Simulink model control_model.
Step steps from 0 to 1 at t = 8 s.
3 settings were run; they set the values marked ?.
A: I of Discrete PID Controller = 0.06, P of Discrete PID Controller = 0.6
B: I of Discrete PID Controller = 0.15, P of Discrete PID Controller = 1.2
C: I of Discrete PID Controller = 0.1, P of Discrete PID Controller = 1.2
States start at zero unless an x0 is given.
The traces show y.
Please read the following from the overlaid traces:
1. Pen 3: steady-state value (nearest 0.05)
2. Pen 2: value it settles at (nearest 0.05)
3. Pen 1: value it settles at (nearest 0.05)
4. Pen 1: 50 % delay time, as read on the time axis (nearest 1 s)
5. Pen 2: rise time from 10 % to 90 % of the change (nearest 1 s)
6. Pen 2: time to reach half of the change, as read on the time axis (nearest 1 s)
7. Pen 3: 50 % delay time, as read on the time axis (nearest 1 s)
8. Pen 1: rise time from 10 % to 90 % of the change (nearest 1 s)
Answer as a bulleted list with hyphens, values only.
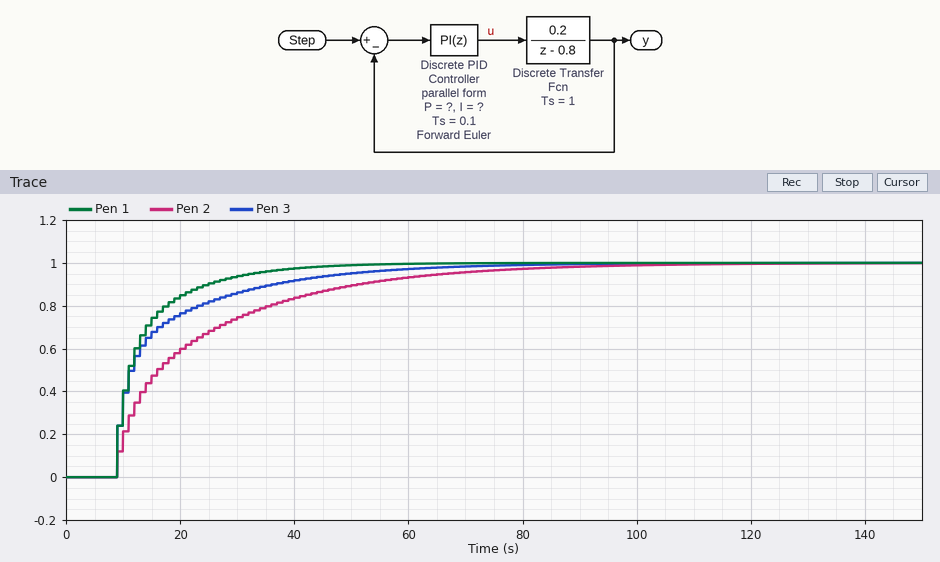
- 1.00
- 1.00
- 1.00
- 11 s
- 42 s
- 16 s
- 12 s
- 16 s
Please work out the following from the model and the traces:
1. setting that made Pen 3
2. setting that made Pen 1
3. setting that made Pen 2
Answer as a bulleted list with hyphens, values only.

- C
- B
- A
